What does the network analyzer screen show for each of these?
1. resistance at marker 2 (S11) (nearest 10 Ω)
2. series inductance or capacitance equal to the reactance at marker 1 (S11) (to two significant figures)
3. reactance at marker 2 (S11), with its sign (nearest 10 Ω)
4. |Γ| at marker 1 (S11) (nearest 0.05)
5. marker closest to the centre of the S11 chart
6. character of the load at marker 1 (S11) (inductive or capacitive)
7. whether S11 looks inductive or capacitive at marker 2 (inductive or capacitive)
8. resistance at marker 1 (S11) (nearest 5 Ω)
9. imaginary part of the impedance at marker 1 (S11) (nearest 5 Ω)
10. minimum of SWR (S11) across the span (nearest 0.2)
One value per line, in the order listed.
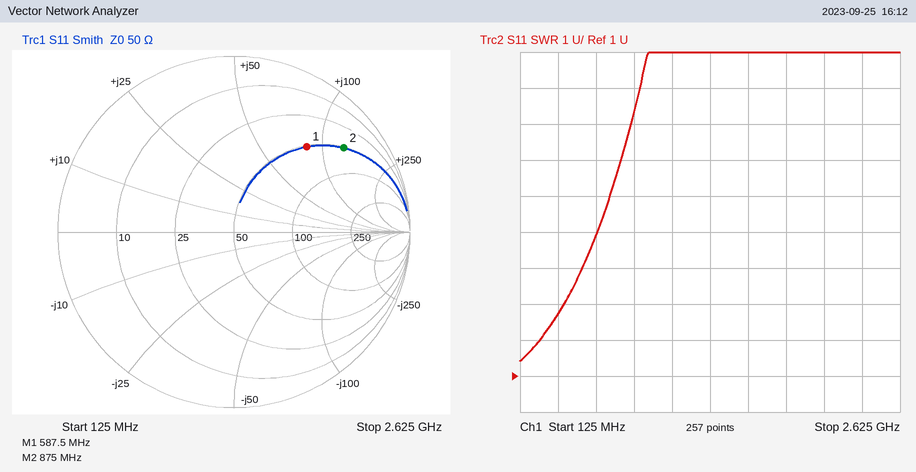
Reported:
50 Ω
23 nH
+130 Ω
0.65
marker 1
inductive
inductive
50 Ω
+85 Ω
1.4
